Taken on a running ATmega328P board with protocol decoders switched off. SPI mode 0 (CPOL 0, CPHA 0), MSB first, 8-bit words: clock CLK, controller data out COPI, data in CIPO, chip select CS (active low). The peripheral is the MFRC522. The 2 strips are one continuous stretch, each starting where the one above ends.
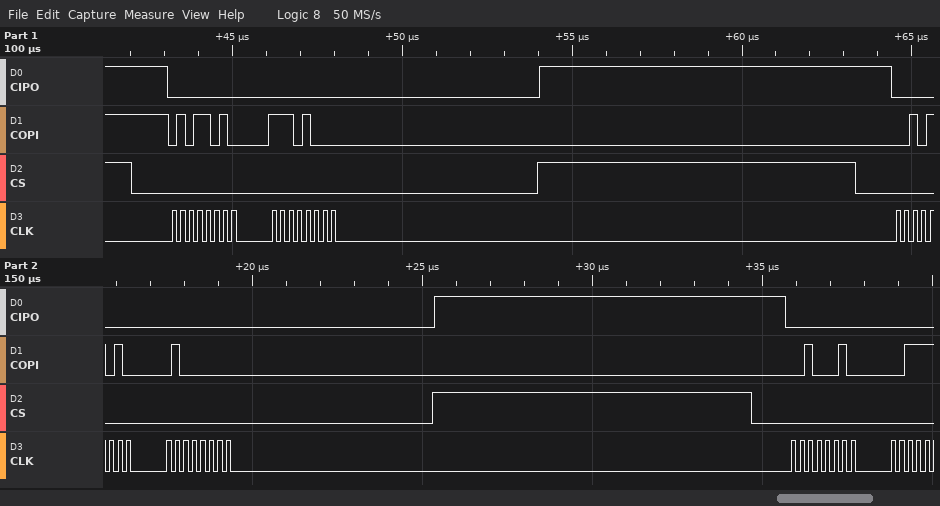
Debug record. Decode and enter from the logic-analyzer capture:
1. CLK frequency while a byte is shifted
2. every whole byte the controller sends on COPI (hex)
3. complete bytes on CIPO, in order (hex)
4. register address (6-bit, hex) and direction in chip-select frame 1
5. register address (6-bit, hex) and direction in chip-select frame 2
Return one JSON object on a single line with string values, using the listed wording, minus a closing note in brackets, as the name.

{"CLK frequency while a byte is shifted": "4 MHz", "every whole byte the controller sends on COPI": "0x5A 0xE8 0x2A 0x40 0x22", "complete bytes on CIPO, in order": "0x00 0x00 0x00 0x00 0x00", "register address (6-bit, hex) and direction in chip-select frame 1": "0x2D write", "register address (6-bit, hex) and direction in chip-select frame 2": "0x15 write"}
